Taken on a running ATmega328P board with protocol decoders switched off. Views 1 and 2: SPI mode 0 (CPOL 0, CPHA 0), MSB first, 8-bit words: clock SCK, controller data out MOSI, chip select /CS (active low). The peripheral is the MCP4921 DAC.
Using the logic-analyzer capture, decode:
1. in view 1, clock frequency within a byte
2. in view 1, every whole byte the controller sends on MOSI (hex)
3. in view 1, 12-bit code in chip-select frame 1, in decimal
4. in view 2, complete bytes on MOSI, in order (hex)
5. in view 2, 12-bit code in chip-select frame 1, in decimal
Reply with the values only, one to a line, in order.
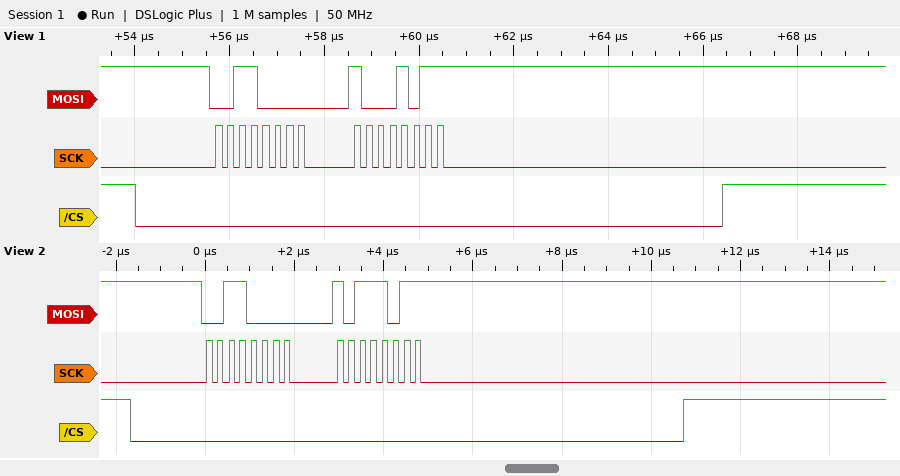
4 MHz
30 8B
139
30 BB
187
